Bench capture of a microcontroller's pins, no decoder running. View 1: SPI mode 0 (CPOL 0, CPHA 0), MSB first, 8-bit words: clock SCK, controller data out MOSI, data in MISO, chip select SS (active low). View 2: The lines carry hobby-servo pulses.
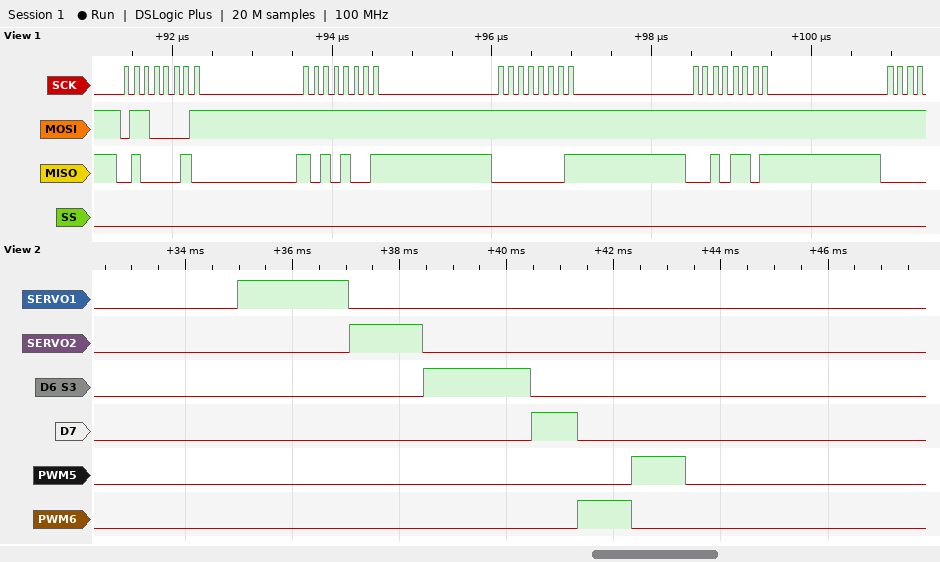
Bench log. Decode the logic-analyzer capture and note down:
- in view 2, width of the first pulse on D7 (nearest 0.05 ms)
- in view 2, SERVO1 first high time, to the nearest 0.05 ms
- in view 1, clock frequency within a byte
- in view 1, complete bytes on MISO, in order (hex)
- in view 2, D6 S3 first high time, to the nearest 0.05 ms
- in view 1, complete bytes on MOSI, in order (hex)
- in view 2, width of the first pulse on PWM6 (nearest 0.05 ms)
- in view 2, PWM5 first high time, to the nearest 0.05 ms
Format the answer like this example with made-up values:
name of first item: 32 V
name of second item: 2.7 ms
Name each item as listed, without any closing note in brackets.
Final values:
in view 2, width of the first pulse on D7: 0.85 ms
in view 2, SERVO1 first high time, to the nearest 0.05 ms: 2.10 ms
in view 1, clock frequency within a byte: 8 MHz
in view 1, complete bytes on MISO, in order: 0x42 0xA9 0x01 0x2D
in view 2, D6 S3 first high time, to the nearest 0.05 ms: 2.00 ms
in view 1, complete bytes on MOSI, in order: 0x61 0xFF 0xFF 0xFF
in view 2, width of the first pulse on PWM6: 1.00 ms
in view 2, PWM5 first high time, to the nearest 0.05 ms: 1.00 ms
